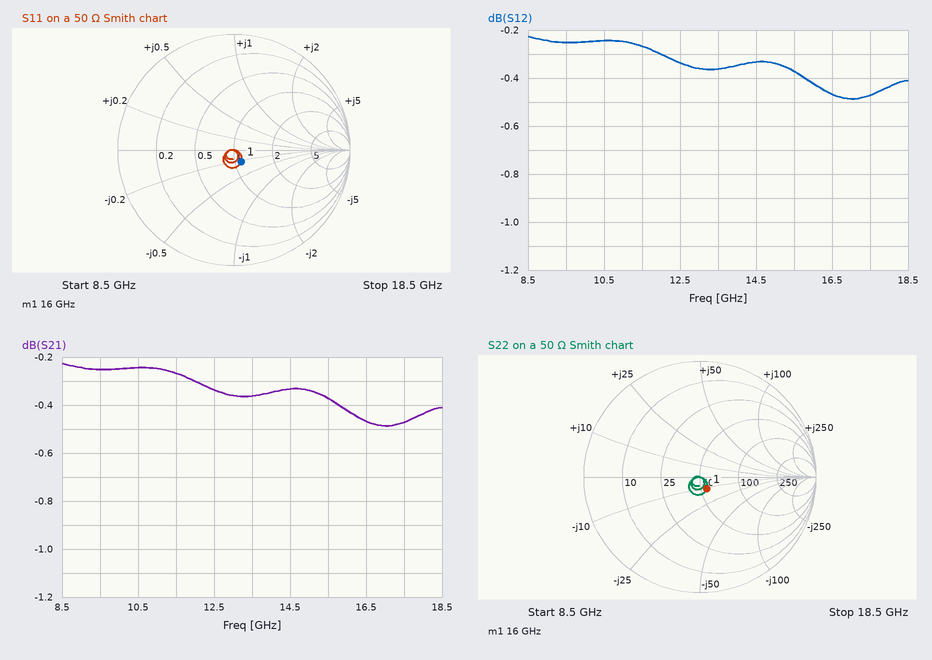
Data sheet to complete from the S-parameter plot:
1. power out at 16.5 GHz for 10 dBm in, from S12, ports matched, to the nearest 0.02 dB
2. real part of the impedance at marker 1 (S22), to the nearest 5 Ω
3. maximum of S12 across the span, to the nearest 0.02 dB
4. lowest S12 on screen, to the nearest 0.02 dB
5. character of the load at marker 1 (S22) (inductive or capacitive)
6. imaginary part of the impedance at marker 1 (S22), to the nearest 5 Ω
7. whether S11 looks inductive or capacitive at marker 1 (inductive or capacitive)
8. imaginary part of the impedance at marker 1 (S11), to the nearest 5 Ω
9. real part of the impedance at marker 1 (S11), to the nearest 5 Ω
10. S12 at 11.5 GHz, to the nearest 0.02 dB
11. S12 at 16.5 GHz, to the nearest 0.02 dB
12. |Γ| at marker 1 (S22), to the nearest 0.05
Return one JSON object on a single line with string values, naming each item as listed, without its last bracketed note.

{"power out at 16.5 GHz for 10 dBm in, from S12, ports matched, to the nearest 0.02 dB": "9.54 dBm", "real part of the impedance at marker 1 (S22), to the nearest 5 Ω": "55 Ω", "maximum of S12 across the span, to the nearest 0.02 dB": "-0.22 dB", "lowest S12 on screen, to the nearest 0.02 dB": "-0.48 dB", "character of the load at marker 1 (S22)": "capacitive", "imaginary part of the impedance at marker 1 (S22), to the nearest 5 Ω": "-10 Ω", "whether S11 looks inductive or capacitive at marker 1": "capacitive", "imaginary part of the impedance at marker 1 (S11), to the nearest 5 Ω": "-10 Ω", "real part of the impedance at marker 1 (S11), to the nearest 5 Ω": "55 Ω", "S12 at 11.5 GHz, to the nearest 0.02 dB": "-0.26 dB", "S12 at 16.5 GHz, to the nearest 0.02 dB": "-0.46 dB", "|Γ| at marker 1 (S22), to the nearest 0.05": "0.10"}
